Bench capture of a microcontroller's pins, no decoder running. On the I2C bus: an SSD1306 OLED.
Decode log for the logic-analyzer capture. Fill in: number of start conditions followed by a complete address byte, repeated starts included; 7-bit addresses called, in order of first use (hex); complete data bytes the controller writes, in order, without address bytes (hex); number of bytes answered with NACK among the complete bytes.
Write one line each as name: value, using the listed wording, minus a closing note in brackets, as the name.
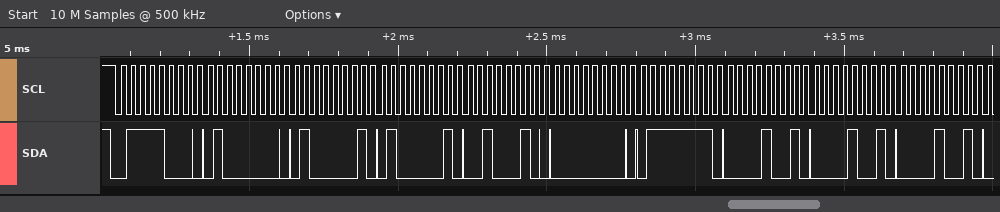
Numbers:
number of start conditions followed by a complete address byte, repeated starts included: 1
7-bit addresses called, in order of first use: 0x3C
complete data bytes the controller writes, in order, without address bytes: 40 41 41 22 00 7F 09 09 09
number of bytes answered with NACK among the complete bytes: 0
